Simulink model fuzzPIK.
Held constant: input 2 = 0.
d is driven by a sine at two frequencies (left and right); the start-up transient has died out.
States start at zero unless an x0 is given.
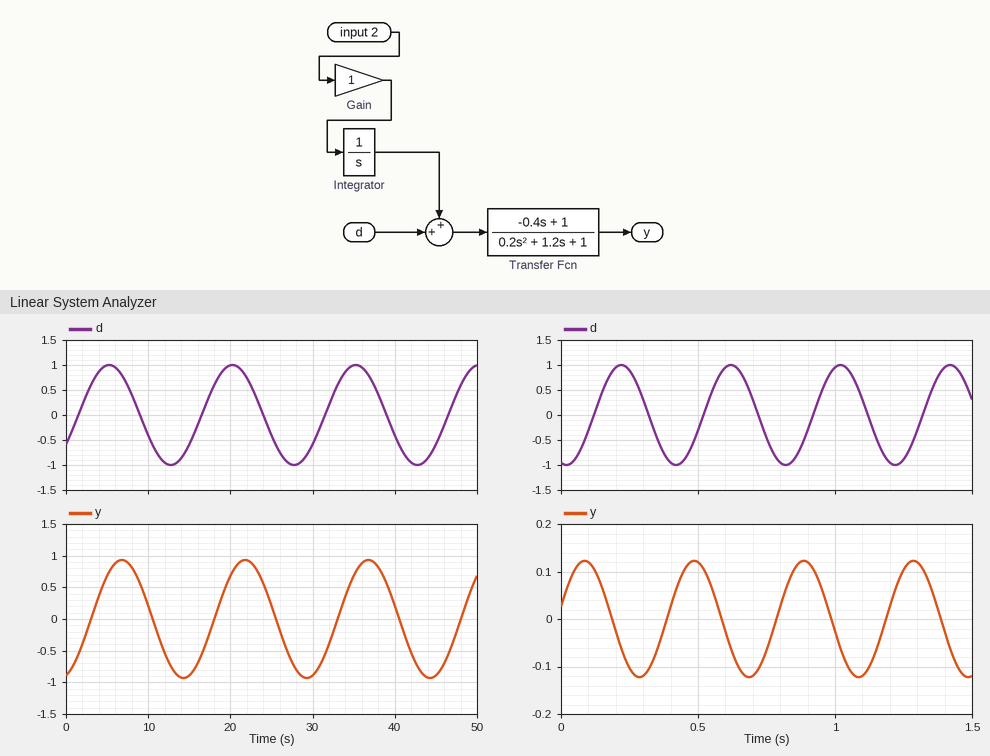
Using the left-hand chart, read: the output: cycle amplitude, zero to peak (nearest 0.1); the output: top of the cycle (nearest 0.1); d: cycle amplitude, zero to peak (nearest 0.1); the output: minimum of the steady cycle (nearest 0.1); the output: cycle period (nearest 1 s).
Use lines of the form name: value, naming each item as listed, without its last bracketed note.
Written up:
the output: cycle amplitude, zero to peak: 0.9
the output: top of the cycle: 0.9
d: cycle amplitude, zero to peak: 1.0
the output: minimum of the steady cycle: -0.9
the output: cycle period: 15 s
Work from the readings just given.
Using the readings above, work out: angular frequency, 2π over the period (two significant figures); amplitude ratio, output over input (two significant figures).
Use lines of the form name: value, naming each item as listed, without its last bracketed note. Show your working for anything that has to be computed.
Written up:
angular frequency, 2π over the period: 2π / 15 = 0.42 rad/s
amplitude ratio, output over input: 0.9 / 1 = 0.90
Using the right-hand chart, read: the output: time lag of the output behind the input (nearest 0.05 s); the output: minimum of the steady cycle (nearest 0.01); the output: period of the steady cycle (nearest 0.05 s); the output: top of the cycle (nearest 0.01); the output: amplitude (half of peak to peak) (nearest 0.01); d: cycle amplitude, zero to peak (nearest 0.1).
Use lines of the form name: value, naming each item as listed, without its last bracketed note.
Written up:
the output: time lag of the output behind the input: 0.25 s
the output: minimum of the steady cycle: -0.12
the output: period of the steady cycle: 0.40 s
the output: top of the cycle: 0.12
the output: amplitude (half of peak to peak): 0.12
d: cycle amplitude, zero to peak: 1.0
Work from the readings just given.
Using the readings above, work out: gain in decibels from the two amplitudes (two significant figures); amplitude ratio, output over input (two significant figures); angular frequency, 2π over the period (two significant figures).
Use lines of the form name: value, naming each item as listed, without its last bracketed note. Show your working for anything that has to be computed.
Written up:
gain in decibels from the two amplitudes: 20 log10(0.12 / 1) = -18 dB
amplitude ratio, output over input: 0.12 / 1 = 0.12
angular frequency, 2π over the period: 2π / 0.4 = 16 rad/s
